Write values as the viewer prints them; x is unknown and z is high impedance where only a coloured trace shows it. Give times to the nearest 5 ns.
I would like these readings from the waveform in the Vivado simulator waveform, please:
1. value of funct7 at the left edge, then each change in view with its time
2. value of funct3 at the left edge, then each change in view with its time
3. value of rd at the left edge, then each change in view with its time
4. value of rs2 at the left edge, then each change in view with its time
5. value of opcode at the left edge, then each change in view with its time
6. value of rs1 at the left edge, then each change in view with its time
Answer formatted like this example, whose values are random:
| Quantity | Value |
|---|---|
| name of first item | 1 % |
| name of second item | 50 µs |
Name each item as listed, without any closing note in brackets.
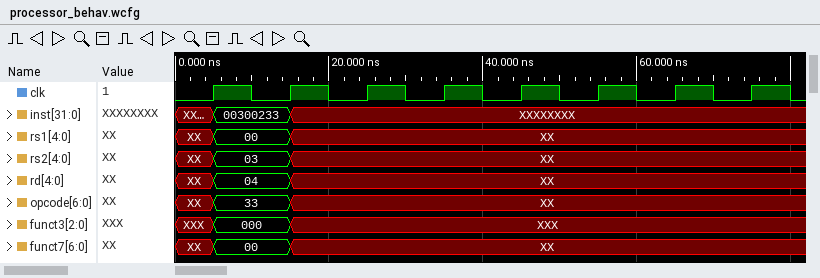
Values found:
| Quantity | Value |
|---|---|
| value of funct7 at the left edge, then each change in view with its time | XX, 00 at 5 ns, XX at 15 ns |
| value of funct3 at the left edge, then each change in view with its time | XXX, 000 at 5 ns, XXX at 15 ns |
| value of rd at the left edge, then each change in view with its time | XX, 04 at 5 ns, XX at 15 ns |
| value of rs2 at the left edge, then each change in view with its time | XX, 03 at 5 ns, XX at 15 ns |
| value of opcode at the left edge, then each change in view with its time | XX, 33 at 5 ns, XX at 15 ns |
| value of rs1 at the left edge, then each change in view with its time | XX, 00 at 5 ns, XX at 15 ns |
